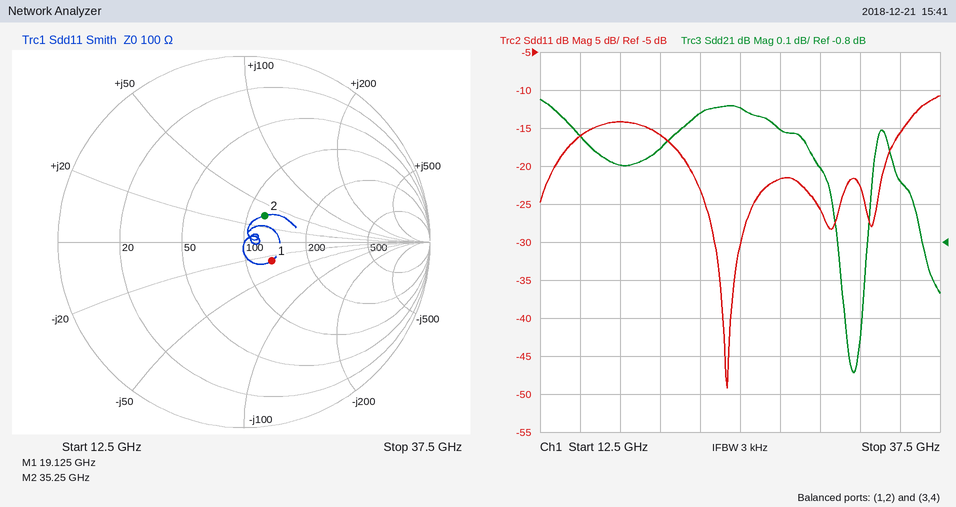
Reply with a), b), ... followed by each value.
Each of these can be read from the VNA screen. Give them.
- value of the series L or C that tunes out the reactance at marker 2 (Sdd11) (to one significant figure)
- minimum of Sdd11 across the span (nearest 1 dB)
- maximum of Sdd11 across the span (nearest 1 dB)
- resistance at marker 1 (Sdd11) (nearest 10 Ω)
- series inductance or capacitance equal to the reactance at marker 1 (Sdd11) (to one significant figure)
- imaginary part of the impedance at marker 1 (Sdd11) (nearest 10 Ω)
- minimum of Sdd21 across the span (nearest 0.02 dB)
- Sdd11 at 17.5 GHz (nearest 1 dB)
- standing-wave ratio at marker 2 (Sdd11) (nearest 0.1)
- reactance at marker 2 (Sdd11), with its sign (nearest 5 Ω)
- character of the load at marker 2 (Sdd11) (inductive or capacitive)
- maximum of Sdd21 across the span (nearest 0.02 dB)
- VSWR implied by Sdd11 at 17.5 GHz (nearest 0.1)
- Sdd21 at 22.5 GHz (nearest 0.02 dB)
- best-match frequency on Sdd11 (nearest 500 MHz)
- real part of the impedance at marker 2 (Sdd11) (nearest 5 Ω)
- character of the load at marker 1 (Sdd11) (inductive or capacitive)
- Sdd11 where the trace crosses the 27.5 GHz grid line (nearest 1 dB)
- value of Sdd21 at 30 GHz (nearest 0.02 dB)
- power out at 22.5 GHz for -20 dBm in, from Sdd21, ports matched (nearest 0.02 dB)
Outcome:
a) 100 fF
b) -49 dB
c) -11 dB
d) 130 Ω
e) 300 fF
f) -30 Ω
g) -1.14 dB
h) -14 dB
i) 1.4
j) +35 Ω
k) inductive
l) -0.42 dB
m) 1.5
n) -0.46 dB
o) 24.0 GHz
p) 120 Ω
q) capacitive
r) -22 dB
s) -0.60 dB
t) -20.46 dBm
